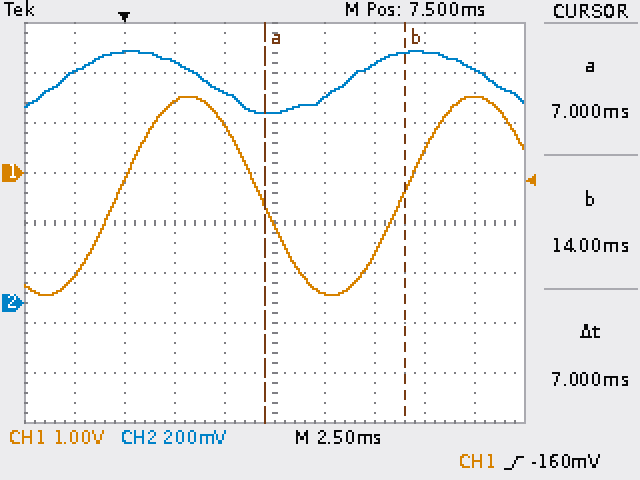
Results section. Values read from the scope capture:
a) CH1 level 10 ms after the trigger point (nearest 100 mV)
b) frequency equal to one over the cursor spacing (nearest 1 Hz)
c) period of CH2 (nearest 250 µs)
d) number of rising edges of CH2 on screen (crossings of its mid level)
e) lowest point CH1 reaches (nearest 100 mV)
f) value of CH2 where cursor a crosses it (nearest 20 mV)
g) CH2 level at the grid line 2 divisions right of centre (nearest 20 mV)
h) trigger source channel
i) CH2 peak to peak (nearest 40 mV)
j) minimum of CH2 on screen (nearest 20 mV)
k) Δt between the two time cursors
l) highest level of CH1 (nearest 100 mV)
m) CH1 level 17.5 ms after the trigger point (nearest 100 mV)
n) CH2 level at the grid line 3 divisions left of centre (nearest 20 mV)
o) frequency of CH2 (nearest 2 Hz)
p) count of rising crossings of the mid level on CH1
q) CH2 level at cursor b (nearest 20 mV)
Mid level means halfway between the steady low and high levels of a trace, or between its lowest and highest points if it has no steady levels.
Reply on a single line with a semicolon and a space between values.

-2.4 V; 143 Hz; 14.25 ms; 2; -2.4 V; 760 mV; 960 mV; CH1; 240 mV; 760 mV; 7 ms; 1.5 V; 1.5 V; 1.00 V; 70 Hz; 2; 1.00 V
